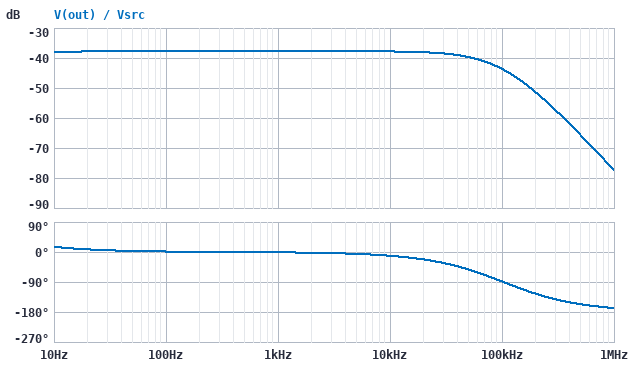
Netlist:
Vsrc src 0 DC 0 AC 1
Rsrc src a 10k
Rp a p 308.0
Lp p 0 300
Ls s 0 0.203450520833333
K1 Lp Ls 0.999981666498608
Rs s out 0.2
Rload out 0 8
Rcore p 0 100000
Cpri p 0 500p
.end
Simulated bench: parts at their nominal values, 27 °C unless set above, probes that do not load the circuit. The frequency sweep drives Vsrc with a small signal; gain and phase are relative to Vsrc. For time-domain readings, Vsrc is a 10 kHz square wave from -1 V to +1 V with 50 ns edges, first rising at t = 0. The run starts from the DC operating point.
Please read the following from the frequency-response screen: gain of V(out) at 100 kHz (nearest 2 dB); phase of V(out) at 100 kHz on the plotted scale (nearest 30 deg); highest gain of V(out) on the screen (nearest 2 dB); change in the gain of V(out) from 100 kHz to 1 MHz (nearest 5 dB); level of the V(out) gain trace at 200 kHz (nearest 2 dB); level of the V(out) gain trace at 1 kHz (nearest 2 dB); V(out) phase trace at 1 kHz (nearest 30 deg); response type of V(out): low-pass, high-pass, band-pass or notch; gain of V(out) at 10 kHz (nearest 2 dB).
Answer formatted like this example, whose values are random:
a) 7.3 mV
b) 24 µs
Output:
a) -44 dB
b) -90 deg
c) -38 dB
d) -35 dB
e) -52 dB
f) -38 dB
g) 0 deg
h) low-pass
i) -38 dB
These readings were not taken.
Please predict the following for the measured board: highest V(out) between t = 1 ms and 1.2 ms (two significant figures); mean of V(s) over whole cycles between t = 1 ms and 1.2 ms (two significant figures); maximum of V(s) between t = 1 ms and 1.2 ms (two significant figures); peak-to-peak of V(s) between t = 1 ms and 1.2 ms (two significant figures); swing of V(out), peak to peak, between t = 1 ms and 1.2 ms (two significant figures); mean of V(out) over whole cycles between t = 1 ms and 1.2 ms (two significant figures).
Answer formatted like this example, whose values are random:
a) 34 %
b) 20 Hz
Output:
a) 26 mV
b) 13 mV
c) 26 mV
d) 27 mV
e) 26 mV
f) 13 mV
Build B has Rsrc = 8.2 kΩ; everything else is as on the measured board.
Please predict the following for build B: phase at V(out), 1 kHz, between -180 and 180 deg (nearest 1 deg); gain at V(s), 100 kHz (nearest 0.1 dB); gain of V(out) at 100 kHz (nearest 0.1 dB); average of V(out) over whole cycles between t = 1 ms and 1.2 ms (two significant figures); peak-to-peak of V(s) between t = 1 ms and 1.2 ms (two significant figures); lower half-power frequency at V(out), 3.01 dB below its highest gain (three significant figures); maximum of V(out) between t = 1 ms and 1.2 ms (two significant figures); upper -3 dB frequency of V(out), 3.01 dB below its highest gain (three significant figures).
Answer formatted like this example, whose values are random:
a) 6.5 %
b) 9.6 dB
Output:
a) -1 deg
b) -42.1 dB
c) -42.3 dB
d) 14 mV
e) 29 mV
f) 2.52 Hz
g) 28 mV
h) 70.0 kHz
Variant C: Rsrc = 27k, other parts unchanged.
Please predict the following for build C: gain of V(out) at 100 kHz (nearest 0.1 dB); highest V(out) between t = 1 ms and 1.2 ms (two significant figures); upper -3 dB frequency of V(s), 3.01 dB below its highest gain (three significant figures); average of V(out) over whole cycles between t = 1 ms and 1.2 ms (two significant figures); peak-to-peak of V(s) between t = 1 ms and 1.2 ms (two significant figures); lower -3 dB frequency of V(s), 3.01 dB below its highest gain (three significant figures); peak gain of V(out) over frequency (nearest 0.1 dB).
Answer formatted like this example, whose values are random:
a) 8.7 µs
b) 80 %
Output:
a) -51.4 dB
b) 14 mV
c) 46.7 kHz
d) 7.0 mV
e) 15 mV
f) 4.10 Hz
g) -42.9 dB
